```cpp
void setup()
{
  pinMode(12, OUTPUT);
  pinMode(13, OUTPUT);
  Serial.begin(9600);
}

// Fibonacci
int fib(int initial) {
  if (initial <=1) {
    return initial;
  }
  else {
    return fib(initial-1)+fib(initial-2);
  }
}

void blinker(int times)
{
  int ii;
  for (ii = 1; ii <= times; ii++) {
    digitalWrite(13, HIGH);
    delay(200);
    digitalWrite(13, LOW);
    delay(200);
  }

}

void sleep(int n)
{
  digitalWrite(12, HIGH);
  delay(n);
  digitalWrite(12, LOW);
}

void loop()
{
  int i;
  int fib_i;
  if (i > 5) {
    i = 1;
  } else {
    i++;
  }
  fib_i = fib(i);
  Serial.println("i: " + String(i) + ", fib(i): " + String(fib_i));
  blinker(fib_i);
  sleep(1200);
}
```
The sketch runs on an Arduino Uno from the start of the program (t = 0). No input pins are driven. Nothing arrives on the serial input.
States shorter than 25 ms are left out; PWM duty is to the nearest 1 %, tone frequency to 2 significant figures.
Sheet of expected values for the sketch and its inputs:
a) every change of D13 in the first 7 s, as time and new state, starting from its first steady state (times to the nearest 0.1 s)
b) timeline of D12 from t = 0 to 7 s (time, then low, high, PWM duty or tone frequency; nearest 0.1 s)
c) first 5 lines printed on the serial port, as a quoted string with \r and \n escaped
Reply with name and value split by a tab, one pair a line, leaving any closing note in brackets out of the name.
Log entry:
every change of D13 in the first 7 s, as time and new state, starting from its first steady state	0 s high; 0.2 s low; 1.6 s high; 1.8 s low; 3.2 s high; 3.4 s low; 4.8 s high; 5 s low; 6.4 s high; 6.6 s low
timeline of D12 from t = 0 to 7 s	0 s low; 0.4 s high; 1.6 s low; 2 s high; 3.2 s low; 3.6 s high; 4.8 s low; 5.2 s high; 6.4 s low; 6.8 s high
first 5 lines printed on the serial port, as a quoted string with \r and \n escaped	"i: 1, fib(i): 1\r\ni: 1, fib(i): 1\r\ni: 1, fib(i): 1\r\ni: 1, fib(i): 1\r\ni: 1, fib(i): 1\r\n"
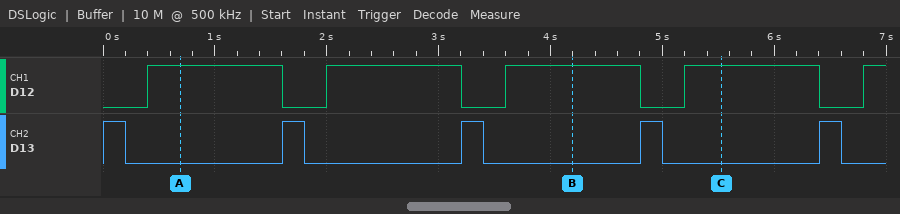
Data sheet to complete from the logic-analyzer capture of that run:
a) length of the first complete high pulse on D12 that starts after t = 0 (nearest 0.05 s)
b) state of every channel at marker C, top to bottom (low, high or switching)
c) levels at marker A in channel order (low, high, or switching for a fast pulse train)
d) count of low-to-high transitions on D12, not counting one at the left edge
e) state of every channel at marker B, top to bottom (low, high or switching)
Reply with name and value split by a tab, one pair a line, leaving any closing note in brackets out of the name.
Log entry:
length of the first complete high pulse on D12 that starts after t = 0	1.20 s
state of every channel at marker C, top to bottom	D12 high, D13 low
levels at marker A in channel order	D12 high, D13 low
count of low-to-high transitions on D12, not counting one at the left edge	5
state of every channel at marker B, top to bottom	D12 high, D13 low
